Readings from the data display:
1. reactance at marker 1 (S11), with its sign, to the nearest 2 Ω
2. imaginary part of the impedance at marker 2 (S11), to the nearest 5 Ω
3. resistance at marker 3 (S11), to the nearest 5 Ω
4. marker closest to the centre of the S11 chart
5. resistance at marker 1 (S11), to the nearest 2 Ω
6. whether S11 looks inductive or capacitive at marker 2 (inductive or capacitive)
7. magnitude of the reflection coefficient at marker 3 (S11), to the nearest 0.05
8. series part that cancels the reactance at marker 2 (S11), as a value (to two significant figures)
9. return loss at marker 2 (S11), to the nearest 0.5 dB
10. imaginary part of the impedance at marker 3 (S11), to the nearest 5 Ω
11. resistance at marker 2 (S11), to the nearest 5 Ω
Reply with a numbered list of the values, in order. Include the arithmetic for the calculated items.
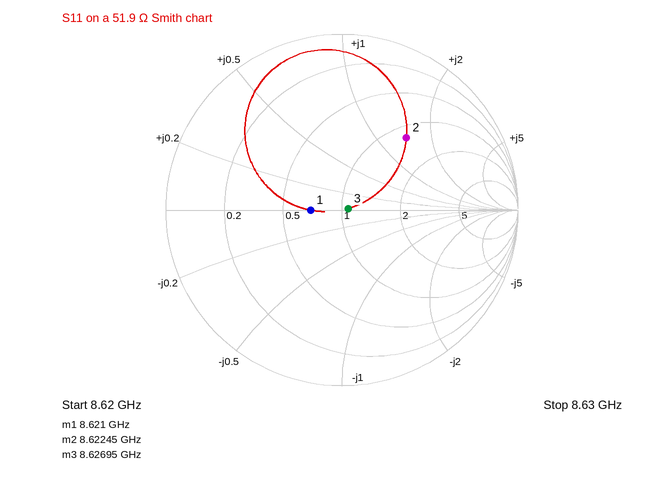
1. 0 Ω
2. +75 Ω
3. 55 Ω
4. marker 3
5. 36 Ω
6. inductive
7. 0.05
8. C = 1/(2π × 8.62245 GHz × 75 Ω) ≈ 246 fF, so 250 fF to two significant figures
9. 5.0 dB
10. 0 Ω
11. 65 Ω
